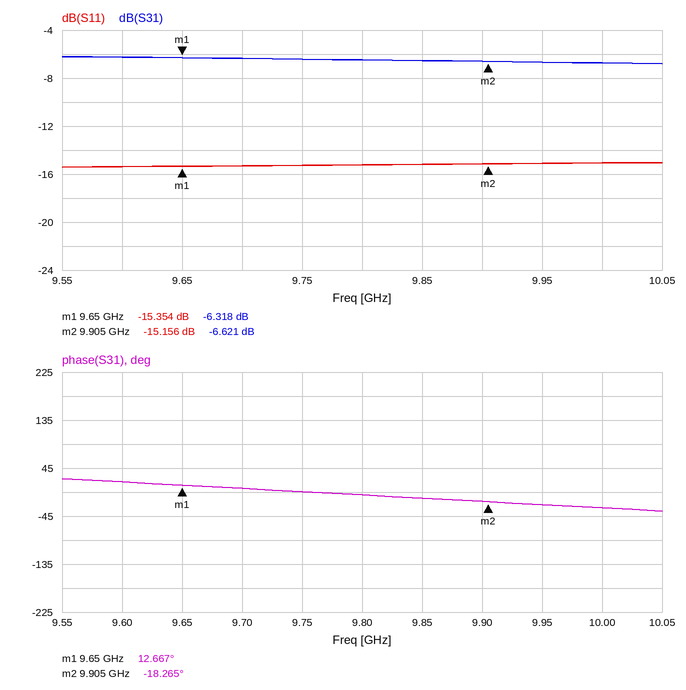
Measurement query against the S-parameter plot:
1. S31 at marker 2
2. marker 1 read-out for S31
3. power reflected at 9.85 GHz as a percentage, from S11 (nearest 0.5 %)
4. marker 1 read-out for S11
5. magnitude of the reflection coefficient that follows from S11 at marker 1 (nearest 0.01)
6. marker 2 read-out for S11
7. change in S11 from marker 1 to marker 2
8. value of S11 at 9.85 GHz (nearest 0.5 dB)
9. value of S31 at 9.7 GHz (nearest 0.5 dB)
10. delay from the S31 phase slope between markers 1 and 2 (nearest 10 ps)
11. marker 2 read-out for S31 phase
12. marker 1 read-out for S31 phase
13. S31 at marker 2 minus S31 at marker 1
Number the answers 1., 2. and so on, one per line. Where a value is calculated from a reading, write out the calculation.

1. -6.621 dB
2. -6.318 dB
3. 10^(-15/10) ≈ 3.16 %, so 3.0 % to the nearest 0.5 %
4. -15.354 dB
5. 10^(-15.354/20) ≈ 0.17
6. -15.156 dB
7. -15.156 − (-15.354) = 0.198 dB
8. -15.0 dB
9. -6.5 dB
10. −(-18.265° − (12.667°))/(360° × 255 MHz) ≈ 337 ps, so 340 ps to the nearest 10 ps
11. -18.265°
12. 12.667°
13. -6.621 − (-6.318) = -0.303 dB
